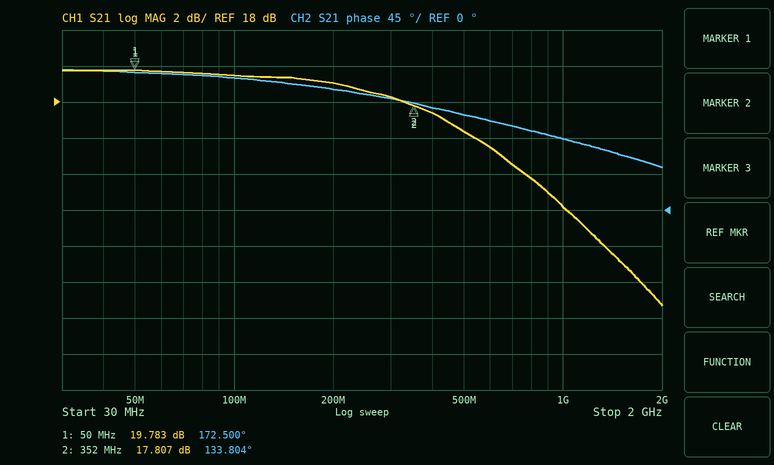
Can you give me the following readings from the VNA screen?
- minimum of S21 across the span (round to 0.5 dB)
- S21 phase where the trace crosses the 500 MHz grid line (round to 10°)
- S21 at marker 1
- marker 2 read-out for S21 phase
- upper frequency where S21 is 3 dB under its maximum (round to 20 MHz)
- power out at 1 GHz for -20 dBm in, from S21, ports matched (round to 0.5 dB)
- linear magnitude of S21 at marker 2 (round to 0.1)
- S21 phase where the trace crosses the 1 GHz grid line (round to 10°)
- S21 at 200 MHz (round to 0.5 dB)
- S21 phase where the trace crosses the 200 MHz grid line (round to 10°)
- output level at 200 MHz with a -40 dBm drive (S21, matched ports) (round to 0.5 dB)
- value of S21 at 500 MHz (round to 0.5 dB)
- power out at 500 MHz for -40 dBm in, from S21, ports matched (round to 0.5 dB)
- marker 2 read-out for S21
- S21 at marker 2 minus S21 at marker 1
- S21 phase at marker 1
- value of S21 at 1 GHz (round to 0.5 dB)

6.5 dB
120°
19.783 dB
133.804°
460 MHz
-8.0 dBm
7.8
90°
19.0 dB
150°
-21.0 dBm
16.5 dB
-23.5 dBm
17.807 dB
-1.976 dB
172.500°
12.0 dB
